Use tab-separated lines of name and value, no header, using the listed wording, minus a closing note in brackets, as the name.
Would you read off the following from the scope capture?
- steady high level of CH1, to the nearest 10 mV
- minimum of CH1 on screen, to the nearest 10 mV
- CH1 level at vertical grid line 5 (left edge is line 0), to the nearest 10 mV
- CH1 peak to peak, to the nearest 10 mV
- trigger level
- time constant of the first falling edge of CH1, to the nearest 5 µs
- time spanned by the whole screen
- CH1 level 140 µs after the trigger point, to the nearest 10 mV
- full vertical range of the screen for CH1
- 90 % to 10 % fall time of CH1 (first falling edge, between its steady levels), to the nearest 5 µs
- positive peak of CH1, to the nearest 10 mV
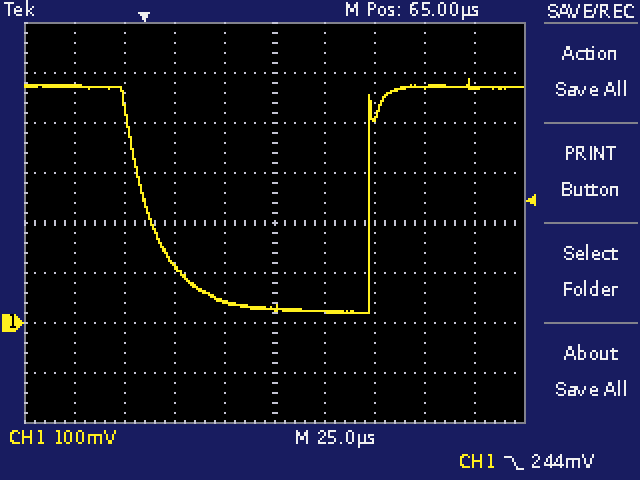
steady high level of CH1, to the nearest 10 mV	470 mV
minimum of CH1 on screen, to the nearest 10 mV	20 mV
CH1 level at vertical grid line 5 (left edge is line 0), to the nearest 10 mV	30 mV
CH1 peak to peak, to the nearest 10 mV	470 mV
trigger level	244 mV
time constant of the first falling edge of CH1, to the nearest 5 µs	15 µs
time spanned by the whole screen	250 µs
CH1 level 140 µs after the trigger point, to the nearest 10 mV	470 mV
full vertical range of the screen for CH1	800 mV
90 % to 10 % fall time of CH1 (first falling edge, between its steady levels), to the nearest 5 µs	35 µs
positive peak of CH1, to the nearest 10 mV	490 mV
